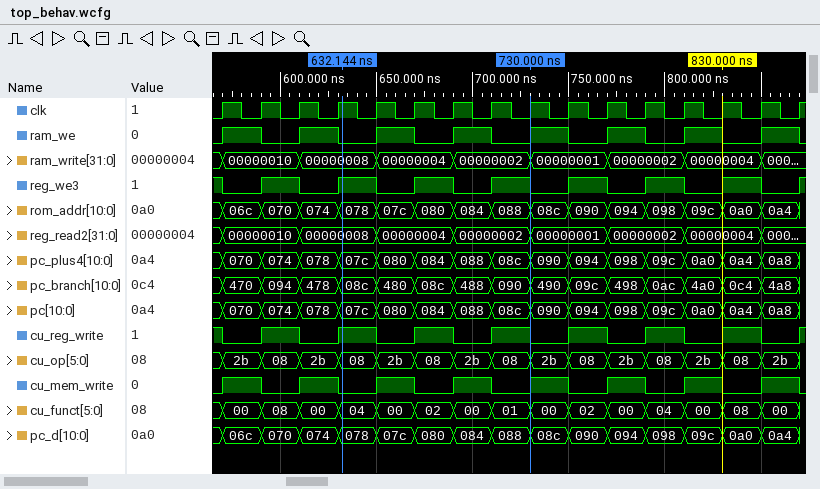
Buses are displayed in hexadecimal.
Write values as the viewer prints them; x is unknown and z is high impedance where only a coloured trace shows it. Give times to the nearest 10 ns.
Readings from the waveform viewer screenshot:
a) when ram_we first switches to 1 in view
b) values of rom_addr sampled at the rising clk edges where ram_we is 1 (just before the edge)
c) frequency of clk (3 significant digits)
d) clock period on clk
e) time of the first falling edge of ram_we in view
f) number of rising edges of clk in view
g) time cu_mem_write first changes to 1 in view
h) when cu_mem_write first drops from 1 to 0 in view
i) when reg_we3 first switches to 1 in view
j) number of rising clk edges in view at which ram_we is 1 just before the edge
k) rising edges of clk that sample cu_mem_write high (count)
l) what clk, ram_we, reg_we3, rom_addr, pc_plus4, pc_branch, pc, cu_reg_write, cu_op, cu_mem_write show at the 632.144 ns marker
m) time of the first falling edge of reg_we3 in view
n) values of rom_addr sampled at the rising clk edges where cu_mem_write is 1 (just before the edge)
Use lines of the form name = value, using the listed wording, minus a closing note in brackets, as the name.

when ram_we first switches to 1 in view = 570 ns
values of rom_addr sampled at the rising clk edges where ram_we is 1 = 06c, 074, 07c, 084, 08c, 094, 09c, 0a4
frequency of clk = 50.0 MHz
clock period on clk = 20 ns
time of the first falling edge of ram_we in view = 590 ns
number of rising edges of clk in view = 16
time cu_mem_write first changes to 1 in view = 570 ns
when cu_mem_write first drops from 1 to 0 in view = 590 ns
when reg_we3 first switches to 1 in view = 590 ns
number of rising clk edges in view at which ram_we is 1 just before the edge = 8
rising edges of clk that sample cu_mem_write high = 8
what clk, ram_we, reg_we3, rom_addr, pc_plus4, pc_branch, pc, cu_reg_write, cu_op, cu_mem_write show at the 632.144 ns marker = clk=1, ram_we=0, reg_we3=1, rom_addr=078, pc_plus4=07c, pc_branch=08c, pc=07c, cu_reg_write=1, cu_op=08, cu_mem_write=0
time of the first falling edge of reg_we3 in view = 570 ns
values of rom_addr sampled at the rising clk edges where cu_mem_write is 1 = 06c, 074, 07c, 084, 08c, 094, 09c, 0a4
